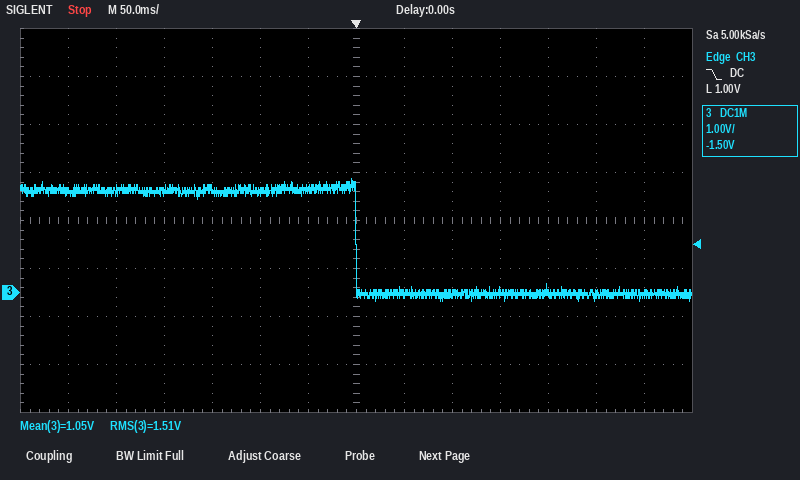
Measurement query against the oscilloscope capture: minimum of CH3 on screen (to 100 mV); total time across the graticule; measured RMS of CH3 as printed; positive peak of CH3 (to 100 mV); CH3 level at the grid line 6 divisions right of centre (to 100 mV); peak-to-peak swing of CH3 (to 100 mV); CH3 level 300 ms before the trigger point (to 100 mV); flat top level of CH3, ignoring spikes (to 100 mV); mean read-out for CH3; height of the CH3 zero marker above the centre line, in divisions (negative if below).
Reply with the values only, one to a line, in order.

-200 mV
700 ms
1.51 V
2.4 V
0.0 V
2.6 V
2.1 V
2.1 V
1.05 V
-1.5 div
